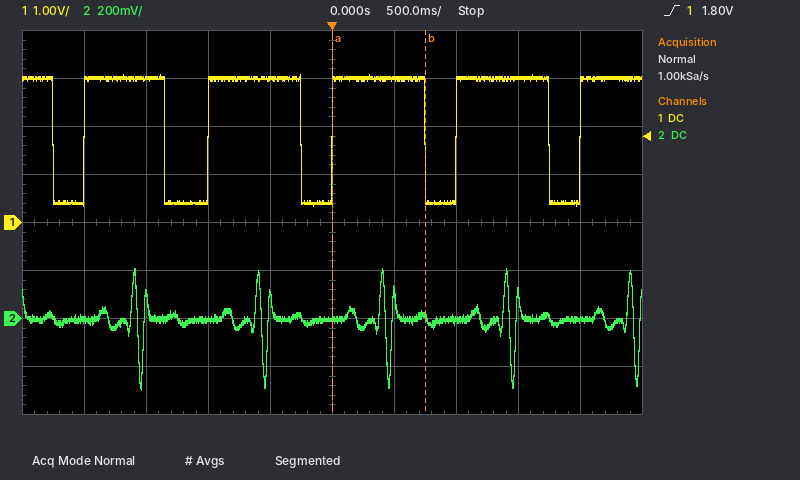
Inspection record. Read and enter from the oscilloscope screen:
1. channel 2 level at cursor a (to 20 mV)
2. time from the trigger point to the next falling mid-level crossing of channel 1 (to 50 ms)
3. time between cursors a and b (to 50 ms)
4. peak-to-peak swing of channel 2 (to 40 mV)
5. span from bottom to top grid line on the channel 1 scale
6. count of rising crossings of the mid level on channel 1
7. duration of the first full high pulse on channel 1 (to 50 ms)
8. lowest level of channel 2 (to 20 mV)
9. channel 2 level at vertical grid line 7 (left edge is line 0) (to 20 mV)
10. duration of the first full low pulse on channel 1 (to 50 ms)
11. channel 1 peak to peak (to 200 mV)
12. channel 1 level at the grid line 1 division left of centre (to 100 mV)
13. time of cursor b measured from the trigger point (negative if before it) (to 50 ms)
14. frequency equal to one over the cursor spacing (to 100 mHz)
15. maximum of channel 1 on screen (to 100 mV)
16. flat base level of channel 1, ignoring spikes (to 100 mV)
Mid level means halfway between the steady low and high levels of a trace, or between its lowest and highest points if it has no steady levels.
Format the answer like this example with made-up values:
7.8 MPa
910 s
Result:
0 mV
750 ms
750 ms
520 mV
8 V
5
650 ms
-300 mV
0 mV
250 ms
2.8 V
3.0 V
+750 ms
1.3 Hz
3.1 V
400 mV
